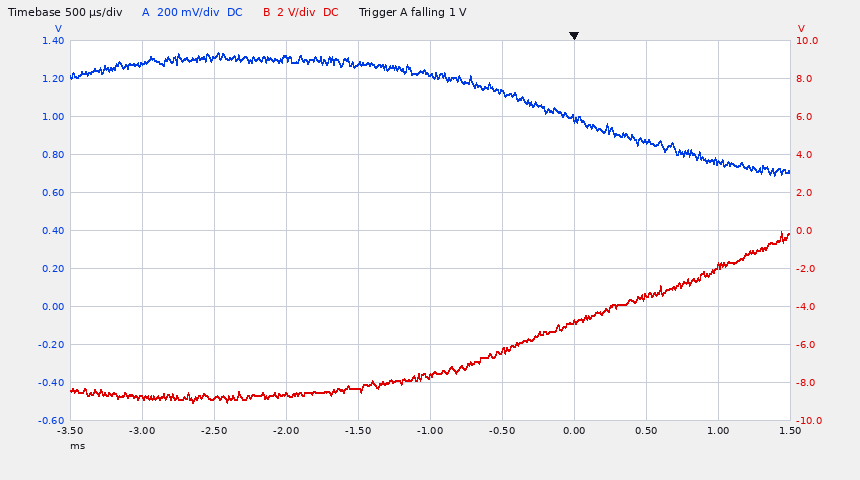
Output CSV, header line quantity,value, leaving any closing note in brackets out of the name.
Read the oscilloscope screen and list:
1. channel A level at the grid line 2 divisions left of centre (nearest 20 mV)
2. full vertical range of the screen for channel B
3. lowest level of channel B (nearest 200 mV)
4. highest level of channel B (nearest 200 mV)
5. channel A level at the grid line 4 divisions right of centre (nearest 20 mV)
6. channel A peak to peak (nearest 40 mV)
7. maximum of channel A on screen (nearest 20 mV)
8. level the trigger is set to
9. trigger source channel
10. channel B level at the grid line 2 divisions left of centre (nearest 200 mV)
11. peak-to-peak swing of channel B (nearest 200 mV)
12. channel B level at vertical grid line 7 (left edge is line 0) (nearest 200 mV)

quantity,value
channel A level at the grid line 2 divisions left of centre,1.30 V
full vertical range of the screen for channel B,20 V
lowest level of channel B,-9.0 V
highest level of channel B,0.0 V
channel A level at the grid line 4 divisions right of centre,760 mV
channel A peak to peak,640 mV
maximum of channel A on screen,1.34 V
level the trigger is set to,1 V
trigger source channel,channel A
channel B level at the grid line 2 divisions left of centre,-8.6 V
peak-to-peak swing of channel B,9.0 V
channel B level at vertical grid line 7 (left edge is line 0),-4.8 V
